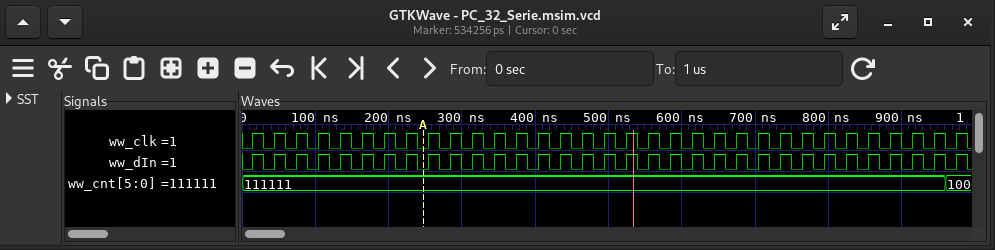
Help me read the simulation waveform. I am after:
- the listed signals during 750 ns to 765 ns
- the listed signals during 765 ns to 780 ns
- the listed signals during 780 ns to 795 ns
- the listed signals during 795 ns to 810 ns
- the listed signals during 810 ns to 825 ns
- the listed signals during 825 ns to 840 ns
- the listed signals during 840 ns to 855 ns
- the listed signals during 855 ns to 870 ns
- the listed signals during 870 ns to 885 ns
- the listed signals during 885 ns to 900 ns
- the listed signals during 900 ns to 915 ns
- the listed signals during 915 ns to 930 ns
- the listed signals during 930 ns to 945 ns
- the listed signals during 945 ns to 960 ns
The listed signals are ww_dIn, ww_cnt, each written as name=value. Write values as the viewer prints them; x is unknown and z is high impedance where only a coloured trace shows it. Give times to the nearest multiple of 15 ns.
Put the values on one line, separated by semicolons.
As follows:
ww_dIn=0, ww_cnt=111111; ww_dIn=1, ww_cnt=111111; ww_dIn=0, ww_cnt=111111; ww_dIn=1, ww_cnt=111111; ww_dIn=0, ww_cnt=111111; ww_dIn=1, ww_cnt=111111; ww_dIn=0, ww_cnt=111111; ww_dIn=1, ww_cnt=111111; ww_dIn=0, ww_cnt=111111; ww_dIn=1, ww_cnt=111111; ww_dIn=0, ww_cnt=111111; ww_dIn=1, ww_cnt=111111; ww_dIn=0, ww_cnt=111111; ww_dIn=1, ww_cnt=111111
